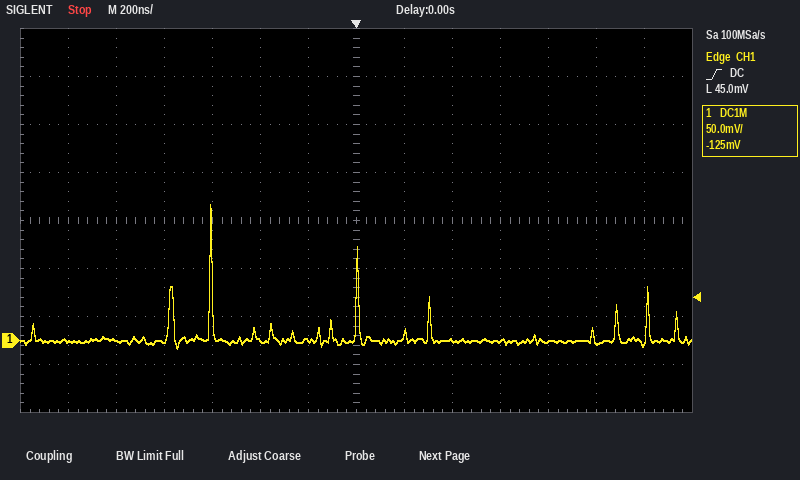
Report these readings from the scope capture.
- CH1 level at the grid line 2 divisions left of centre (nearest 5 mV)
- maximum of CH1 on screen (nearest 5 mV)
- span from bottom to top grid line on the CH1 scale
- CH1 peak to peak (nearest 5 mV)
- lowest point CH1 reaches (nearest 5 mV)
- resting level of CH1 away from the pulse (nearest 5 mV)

0 mV
140 mV
400 mV
150 mV
-10 mV
0 mV
